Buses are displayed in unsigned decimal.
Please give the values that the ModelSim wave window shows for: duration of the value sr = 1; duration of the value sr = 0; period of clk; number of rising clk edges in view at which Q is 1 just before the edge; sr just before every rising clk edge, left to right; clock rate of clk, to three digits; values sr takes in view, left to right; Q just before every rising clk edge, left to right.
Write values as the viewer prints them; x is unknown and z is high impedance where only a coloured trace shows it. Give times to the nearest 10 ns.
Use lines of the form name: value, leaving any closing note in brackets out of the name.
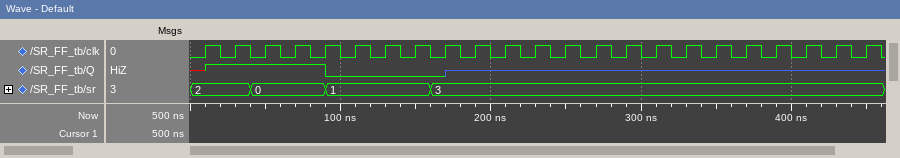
duration of the value sr = 1: 70 ns
duration of the value sr = 0: 50 ns
period of clk: 20 ns
number of rising clk edges in view at which Q is 1 just before the edge: 4
sr just before every rising clk edge, left to right: 2, 2, 0, 0, 0, 1, 1, 1, 3, 3, 3, 3, 3, 3, 3, 3, 3, 3, 3, 3, 3, 3, 3
clock rate of clk, to three digits: 50.0 MHz
values sr takes in view, left to right: 2, 0, 1, 3
Q just before every rising clk edge, left to right: x 1 1 1 1 0 0 0 0 z z z z z z z z z z z z z z
